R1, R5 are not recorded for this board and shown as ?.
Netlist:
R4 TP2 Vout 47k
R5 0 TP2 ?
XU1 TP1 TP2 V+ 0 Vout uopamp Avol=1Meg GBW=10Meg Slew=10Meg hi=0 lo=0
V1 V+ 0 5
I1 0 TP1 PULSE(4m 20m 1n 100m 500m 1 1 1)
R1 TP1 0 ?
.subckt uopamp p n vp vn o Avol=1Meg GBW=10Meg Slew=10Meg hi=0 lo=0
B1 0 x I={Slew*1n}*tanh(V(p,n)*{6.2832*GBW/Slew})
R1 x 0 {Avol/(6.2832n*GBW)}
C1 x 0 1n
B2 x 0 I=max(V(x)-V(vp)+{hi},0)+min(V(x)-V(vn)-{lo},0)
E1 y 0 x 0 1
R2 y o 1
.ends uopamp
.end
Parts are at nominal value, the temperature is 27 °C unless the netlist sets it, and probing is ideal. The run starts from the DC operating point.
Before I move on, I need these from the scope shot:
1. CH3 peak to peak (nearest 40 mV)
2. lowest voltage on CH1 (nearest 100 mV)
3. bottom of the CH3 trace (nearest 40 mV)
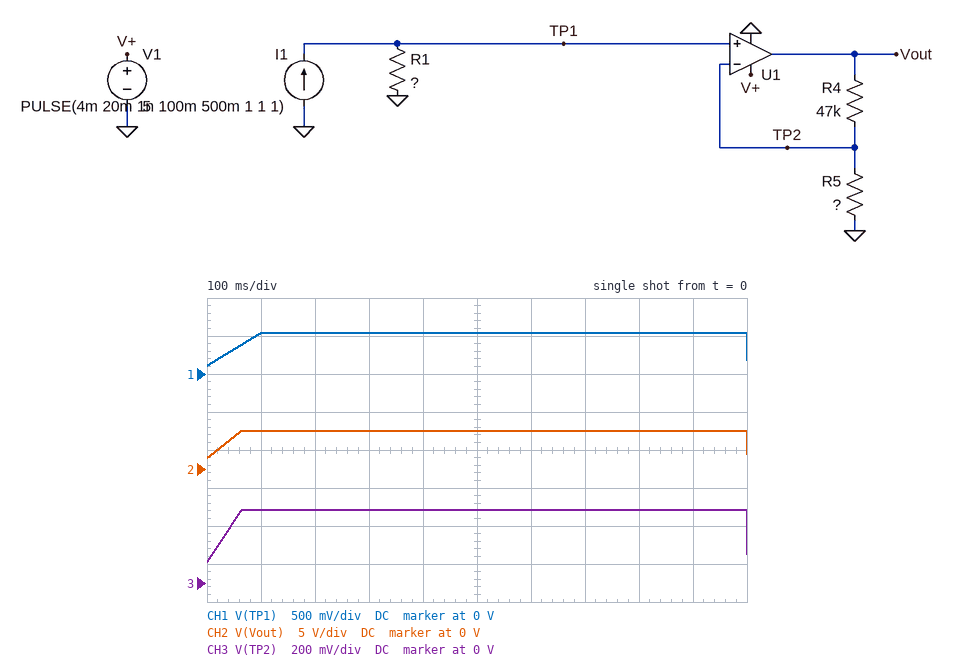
280 mV
100 mV
120 mV
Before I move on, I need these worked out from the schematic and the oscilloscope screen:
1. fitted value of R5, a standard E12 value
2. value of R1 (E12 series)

3.9 kΩ
27 Ω
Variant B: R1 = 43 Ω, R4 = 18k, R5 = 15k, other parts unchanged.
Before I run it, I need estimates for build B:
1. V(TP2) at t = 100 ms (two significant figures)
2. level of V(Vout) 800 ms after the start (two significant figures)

860 mV
1.9 V
